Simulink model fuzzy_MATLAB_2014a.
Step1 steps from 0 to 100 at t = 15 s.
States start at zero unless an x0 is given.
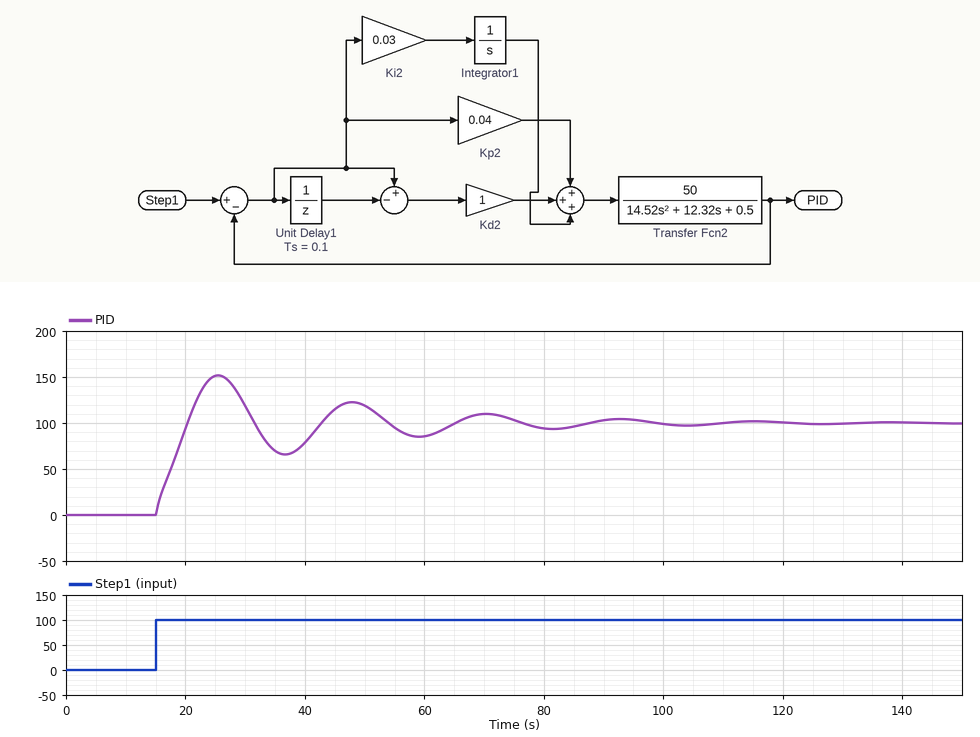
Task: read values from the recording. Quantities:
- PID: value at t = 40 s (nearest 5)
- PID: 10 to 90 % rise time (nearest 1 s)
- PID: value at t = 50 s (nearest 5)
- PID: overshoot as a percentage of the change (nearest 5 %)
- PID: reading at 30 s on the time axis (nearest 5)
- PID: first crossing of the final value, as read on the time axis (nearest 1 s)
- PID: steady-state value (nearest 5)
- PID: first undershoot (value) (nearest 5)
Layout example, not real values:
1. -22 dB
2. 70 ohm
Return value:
1. 80
2. 4 s
3. 120
4. 50 %
5. 120
6. 20 s
7. 100
8. 65
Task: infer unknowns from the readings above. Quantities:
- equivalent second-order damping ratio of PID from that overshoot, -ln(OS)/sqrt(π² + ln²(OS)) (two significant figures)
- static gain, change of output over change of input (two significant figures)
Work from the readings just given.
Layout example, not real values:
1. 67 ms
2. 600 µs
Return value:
1. 0.22
2. 1.0
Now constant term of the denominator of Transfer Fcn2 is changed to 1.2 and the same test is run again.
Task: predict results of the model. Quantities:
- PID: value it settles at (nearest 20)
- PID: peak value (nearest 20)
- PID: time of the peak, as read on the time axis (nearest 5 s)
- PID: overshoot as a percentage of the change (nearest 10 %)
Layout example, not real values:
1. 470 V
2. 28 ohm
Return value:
1. 100
2. 140
3. 25 s
4. 40 %
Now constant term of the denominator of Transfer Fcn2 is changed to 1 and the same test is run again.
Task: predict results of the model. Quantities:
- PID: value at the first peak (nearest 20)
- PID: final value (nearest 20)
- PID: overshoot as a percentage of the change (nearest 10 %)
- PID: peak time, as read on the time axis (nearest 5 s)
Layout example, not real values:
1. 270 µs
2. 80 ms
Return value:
1. 140
2. 100
3. 40 %
4. 25 s
